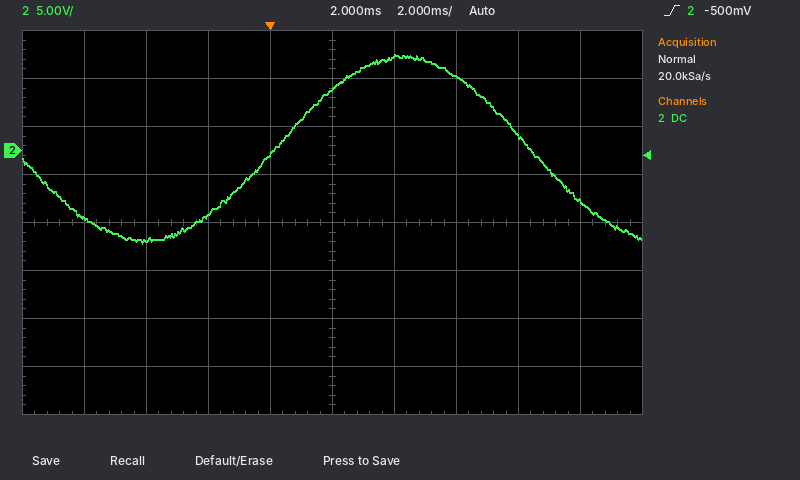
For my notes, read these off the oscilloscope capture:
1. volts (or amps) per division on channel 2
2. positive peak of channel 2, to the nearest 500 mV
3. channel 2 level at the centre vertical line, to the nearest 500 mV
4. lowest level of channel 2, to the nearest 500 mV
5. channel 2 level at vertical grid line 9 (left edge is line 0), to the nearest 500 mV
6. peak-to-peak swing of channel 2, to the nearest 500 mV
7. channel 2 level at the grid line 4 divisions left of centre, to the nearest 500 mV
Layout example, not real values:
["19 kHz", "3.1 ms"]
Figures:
["5 V", "10.0 V", "6.5 V", "-9.5 V", "-5.5 V", "19.5 V", "-7.0 V"]
